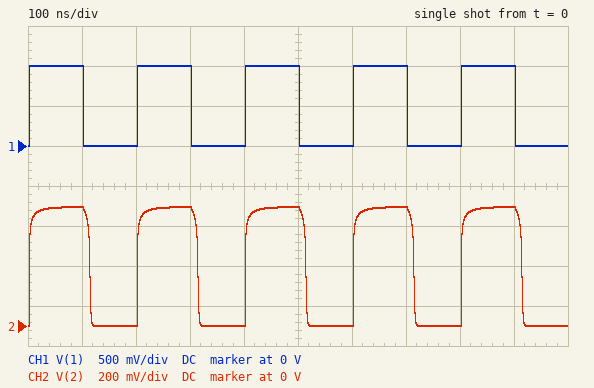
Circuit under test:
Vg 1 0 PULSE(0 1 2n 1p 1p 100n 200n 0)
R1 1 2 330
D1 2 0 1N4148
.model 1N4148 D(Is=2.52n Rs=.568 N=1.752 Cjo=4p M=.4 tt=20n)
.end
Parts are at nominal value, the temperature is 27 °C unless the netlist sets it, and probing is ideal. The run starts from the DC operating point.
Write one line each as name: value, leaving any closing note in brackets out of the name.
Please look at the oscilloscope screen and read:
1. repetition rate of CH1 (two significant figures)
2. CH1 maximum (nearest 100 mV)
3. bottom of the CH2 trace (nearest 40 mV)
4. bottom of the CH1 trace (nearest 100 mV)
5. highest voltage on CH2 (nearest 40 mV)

repetition rate of CH1: 5.0 MHz
CH1 maximum: 1.0 V
bottom of the CH2 trace: 0 V
bottom of the CH1 trace: 0 V
highest voltage on CH2: 600 mV
